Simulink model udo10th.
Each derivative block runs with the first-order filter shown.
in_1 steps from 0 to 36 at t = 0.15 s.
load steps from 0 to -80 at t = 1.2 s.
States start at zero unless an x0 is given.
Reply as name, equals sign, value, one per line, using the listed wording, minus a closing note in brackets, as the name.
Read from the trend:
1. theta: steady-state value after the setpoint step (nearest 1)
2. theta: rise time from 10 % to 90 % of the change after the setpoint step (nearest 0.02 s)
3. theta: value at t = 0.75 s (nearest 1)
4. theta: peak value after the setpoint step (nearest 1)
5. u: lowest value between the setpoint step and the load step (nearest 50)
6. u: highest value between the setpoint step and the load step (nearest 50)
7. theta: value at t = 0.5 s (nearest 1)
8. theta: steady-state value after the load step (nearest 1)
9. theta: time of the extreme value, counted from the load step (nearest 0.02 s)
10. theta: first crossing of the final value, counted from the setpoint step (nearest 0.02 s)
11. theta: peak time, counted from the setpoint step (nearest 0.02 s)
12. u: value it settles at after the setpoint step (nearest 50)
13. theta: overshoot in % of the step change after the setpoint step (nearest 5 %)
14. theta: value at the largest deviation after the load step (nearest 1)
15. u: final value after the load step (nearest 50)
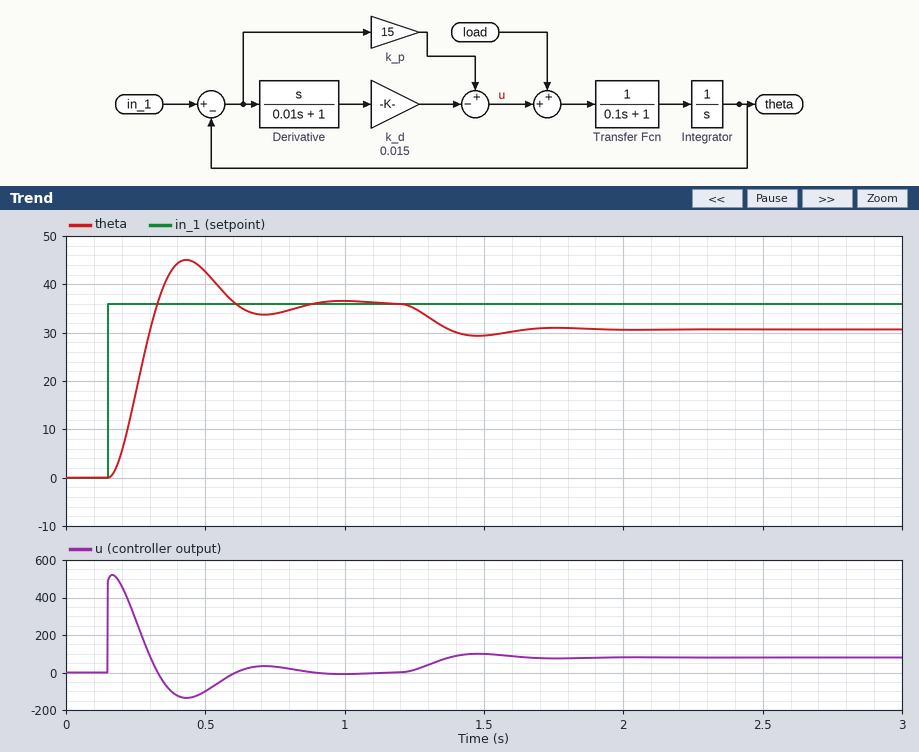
theta: steady-state value after the setpoint step = 36
theta: rise time from 10 % to 90 % of the change after the setpoint step = 0.12 s
theta: value at t = 0.75 s = 34
theta: peak value after the setpoint step = 45
u: lowest value between the setpoint step and the load step = -150
u: highest value between the setpoint step and the load step = 500
theta: value at t = 0.5 s = 43
theta: steady-state value after the load step = 31
theta: time of the extreme value, counted from the load step = 0.28 s
theta: first crossing of the final value, counted from the setpoint step = 0.18 s
theta: peak time, counted from the setpoint step = 0.28 s
u: value it settles at after the setpoint step = 0
theta: overshoot in % of the step change after the setpoint step = 25 %
theta: value at the largest deviation after the load step = 29
u: final value after the load step = 100
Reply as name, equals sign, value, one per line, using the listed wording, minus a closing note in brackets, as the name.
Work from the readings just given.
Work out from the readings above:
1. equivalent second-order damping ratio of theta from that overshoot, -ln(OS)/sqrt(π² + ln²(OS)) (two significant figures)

equivalent second-order damping ratio of theta from that overshoot, -ln(OS)/sqrt(π² + ln²(OS)) = 0.40
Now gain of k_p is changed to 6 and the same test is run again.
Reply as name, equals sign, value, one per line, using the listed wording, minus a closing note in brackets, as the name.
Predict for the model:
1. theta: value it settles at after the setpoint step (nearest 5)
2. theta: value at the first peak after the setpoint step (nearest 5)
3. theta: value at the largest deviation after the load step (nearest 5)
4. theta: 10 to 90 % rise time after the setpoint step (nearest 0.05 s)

theta: value it settles at after the setpoint step = 35
theta: value at the first peak after the setpoint step = 40
theta: value at the largest deviation after the load step = 20
theta: 10 to 90 % rise time after the setpoint step = 0.25 s
